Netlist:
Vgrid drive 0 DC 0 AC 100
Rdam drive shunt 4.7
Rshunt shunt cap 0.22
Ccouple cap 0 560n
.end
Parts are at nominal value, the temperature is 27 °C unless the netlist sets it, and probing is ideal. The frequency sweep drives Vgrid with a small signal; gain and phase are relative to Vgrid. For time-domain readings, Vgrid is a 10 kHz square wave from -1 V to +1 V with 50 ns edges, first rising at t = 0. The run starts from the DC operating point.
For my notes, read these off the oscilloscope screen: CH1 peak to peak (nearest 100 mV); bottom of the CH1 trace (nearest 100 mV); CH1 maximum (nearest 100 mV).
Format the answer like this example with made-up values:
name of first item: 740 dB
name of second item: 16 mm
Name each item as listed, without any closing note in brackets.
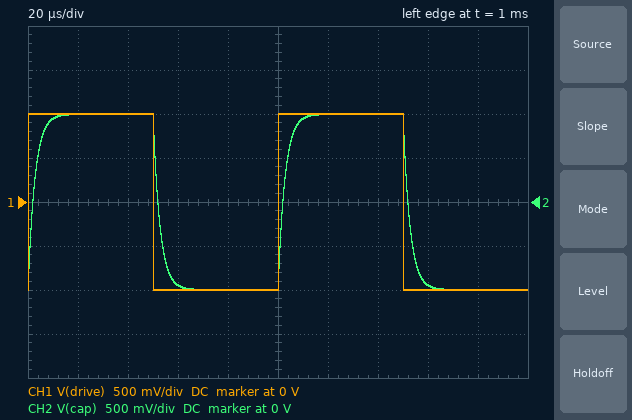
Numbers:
CH1 peak to peak: 2.0 V
bottom of the CH1 trace: -1.0 V
CH1 maximum: 1.0 V
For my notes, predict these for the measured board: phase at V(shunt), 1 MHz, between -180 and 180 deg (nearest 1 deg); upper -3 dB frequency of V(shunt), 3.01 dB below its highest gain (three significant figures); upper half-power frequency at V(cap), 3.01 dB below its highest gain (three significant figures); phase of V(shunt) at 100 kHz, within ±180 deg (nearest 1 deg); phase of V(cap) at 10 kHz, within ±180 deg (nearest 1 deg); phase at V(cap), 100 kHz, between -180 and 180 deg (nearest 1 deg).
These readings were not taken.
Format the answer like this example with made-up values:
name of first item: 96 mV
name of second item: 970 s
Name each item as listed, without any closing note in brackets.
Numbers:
phase at V(shunt), 1 MHz, between -180 and 180 deg: -49 deg
upper -3 dB frequency of V(shunt), 3.01 dB below its highest gain: 57.9 kHz
upper half-power frequency at V(cap), 3.01 dB below its highest gain: 57.8 kHz
phase of V(shunt) at 100 kHz, within ±180 deg: -56 deg
phase of V(cap) at 10 kHz, within ±180 deg: -10 deg
phase at V(cap), 100 kHz, between -180 and 180 deg: -60 deg
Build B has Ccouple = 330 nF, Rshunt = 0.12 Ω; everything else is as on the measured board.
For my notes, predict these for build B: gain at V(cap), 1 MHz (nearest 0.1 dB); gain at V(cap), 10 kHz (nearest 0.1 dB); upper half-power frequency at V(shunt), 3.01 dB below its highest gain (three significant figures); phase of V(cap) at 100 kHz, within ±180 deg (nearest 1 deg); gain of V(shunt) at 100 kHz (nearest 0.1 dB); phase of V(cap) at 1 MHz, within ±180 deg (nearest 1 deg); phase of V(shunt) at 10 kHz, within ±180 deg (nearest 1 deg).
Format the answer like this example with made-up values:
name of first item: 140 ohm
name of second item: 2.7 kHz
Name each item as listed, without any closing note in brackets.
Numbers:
gain at V(cap), 1 MHz: -20.0 dB
gain at V(cap), 10 kHz: 0 dB
upper half-power frequency at V(shunt), 3.01 dB below its highest gain: 100 kHz
phase of V(cap) at 100 kHz, within ±180 deg: -45 deg
gain of V(shunt) at 100 kHz: -3.0 dB
phase of V(cap) at 1 MHz, within ±180 deg: -84 deg
phase of V(shunt) at 10 kHz, within ±180 deg: -6 deg
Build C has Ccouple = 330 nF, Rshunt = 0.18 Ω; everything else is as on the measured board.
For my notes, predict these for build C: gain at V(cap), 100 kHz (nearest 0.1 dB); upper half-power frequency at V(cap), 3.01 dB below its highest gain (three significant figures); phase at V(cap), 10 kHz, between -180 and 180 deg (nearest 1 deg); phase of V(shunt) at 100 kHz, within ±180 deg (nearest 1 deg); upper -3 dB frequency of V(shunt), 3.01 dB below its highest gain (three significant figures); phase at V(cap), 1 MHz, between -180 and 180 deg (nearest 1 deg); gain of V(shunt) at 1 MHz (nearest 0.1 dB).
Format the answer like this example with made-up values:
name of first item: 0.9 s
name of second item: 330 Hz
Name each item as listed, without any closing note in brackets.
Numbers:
gain at V(cap), 100 kHz: -3.1 dB
upper half-power frequency at V(cap), 3.01 dB below its highest gain: 98.8 kHz
phase at V(cap), 10 kHz, between -180 and 180 deg: -6 deg
phase of V(shunt) at 100 kHz, within ±180 deg: -43 deg
upper -3 dB frequency of V(shunt), 3.01 dB below its highest gain: 99.0 kHz
phase at V(cap), 1 MHz, between -180 and 180 deg: -84 deg
gain of V(shunt) at 1 MHz: -19.6 dB
